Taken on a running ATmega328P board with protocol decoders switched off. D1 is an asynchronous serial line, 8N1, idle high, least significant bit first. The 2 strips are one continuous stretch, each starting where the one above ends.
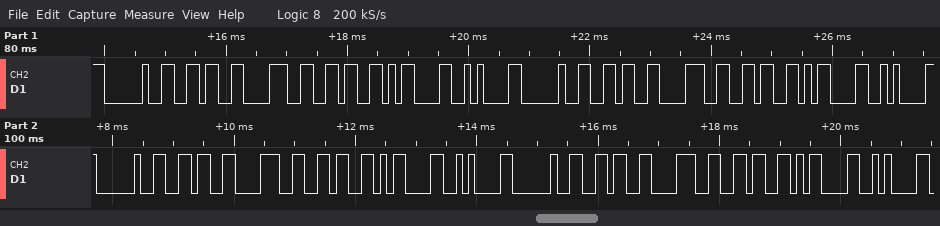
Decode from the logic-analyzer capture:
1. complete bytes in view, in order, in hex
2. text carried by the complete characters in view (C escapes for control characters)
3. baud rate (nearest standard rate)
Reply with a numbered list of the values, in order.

1. 20 36 38 36 0D 0A 20 36 38 36 0D 0A 20 36 38 36 0D 0A 20 36 38 36 0D 0A
2. " 686\r\n 686\r\n 686\r\n 686\r\n"
3. 9600 baud
